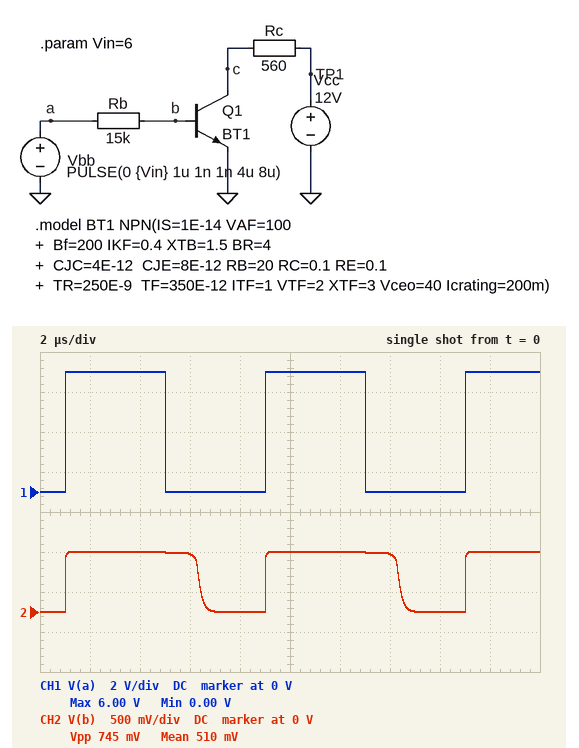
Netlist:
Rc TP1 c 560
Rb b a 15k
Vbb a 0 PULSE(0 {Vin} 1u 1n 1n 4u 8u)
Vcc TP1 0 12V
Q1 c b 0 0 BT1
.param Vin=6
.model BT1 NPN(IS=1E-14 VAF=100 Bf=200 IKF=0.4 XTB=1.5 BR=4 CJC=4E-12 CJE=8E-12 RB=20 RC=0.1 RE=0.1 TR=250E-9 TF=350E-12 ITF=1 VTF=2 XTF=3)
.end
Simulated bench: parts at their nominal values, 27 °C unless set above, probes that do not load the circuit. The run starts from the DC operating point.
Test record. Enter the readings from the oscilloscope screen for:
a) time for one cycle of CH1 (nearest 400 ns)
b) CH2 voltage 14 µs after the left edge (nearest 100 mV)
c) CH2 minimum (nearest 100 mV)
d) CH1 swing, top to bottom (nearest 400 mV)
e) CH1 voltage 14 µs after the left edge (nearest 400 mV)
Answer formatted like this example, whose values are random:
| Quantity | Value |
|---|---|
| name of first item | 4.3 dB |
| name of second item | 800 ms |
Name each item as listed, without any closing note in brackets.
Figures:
| Quantity | Value |
|---|---|
| time for one cycle of CH1 | 8.0 µs |
| CH2 voltage 14 µs after the left edge | 700 mV |
| CH2 minimum | 0 V |
| CH1 swing, top to bottom | 6.0 V |
| CH1 voltage 14 µs after the left edge | 0 V |
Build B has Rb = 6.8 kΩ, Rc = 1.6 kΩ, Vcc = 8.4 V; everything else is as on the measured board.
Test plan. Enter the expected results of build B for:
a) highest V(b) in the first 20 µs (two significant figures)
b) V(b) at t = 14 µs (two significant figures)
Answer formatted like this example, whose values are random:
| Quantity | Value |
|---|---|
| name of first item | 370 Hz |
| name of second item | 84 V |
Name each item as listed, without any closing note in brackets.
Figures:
| Quantity | Value |
|---|---|
| highest V(b) in the first 20 µs | 730 mV |
| V(b) at t = 14 µs | 700 mV |
